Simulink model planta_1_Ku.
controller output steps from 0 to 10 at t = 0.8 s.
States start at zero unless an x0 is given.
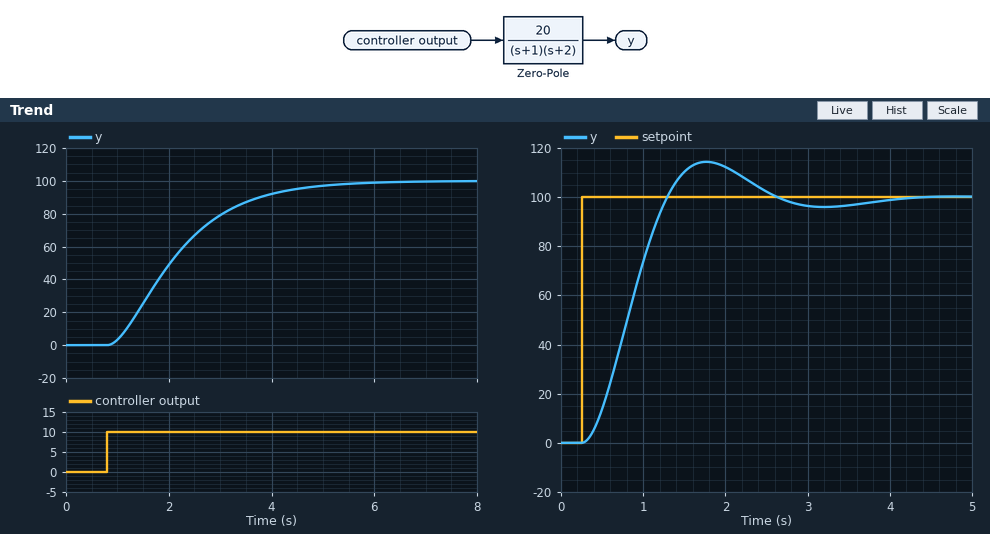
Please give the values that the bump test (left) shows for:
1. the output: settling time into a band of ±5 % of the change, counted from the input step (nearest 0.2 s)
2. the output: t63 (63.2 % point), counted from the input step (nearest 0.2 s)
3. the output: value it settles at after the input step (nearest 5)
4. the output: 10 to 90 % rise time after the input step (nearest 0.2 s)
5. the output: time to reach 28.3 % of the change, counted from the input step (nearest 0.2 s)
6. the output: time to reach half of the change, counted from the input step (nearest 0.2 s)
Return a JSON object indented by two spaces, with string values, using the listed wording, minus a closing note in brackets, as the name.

{
  "the output: settling time into a band of ±5 % of the change, counted from the input step": "3.6 s",
  "the output: t63 (63.2 % point), counted from the input step": "1.6 s",
  "the output: value it settles at after the input step": "100",
  "the output: 10 to 90 % rise time after the input step": "2.6 s",
  "the output: time to reach 28.3 % of the change, counted from the input step": "0.8 s",
  "the output: time to reach half of the change, counted from the input step": "1.2 s"
}
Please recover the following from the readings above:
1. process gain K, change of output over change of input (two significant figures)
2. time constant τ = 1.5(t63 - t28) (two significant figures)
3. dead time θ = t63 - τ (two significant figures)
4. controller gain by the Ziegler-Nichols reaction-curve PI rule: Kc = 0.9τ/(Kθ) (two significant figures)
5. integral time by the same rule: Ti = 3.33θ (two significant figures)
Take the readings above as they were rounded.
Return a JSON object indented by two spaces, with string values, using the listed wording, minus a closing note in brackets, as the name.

{
  "process gain K, change of output over change of input": "10",
  "time constant τ = 1.5(t63 - t28)": "1.2 s",
  "dead time θ = t63 - τ": "0.40 s",
  "controller gain by the Ziegler-Nichols reaction-curve PI rule: Kc = 0.9τ/(Kθ)": "0.27",
  "integral time by the same rule: Ti = 3.33θ": "1.3 s"
}
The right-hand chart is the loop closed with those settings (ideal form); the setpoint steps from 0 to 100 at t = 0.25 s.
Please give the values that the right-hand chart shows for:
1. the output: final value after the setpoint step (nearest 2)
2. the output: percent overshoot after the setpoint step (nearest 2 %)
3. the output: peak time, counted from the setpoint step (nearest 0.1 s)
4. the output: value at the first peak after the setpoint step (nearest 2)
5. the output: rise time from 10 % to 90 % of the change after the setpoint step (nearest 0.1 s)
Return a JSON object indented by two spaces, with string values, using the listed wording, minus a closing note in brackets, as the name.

{
  "the output: final value after the setpoint step": "100",
  "the output: percent overshoot after the setpoint step": "14 %",
  "the output: peak time, counted from the setpoint step": "1.5 s",
  "the output: value at the first peak after the setpoint step": "114",
  "the output: rise time from 10 % to 90 % of the change after the setpoint step": "0.7 s"
}
